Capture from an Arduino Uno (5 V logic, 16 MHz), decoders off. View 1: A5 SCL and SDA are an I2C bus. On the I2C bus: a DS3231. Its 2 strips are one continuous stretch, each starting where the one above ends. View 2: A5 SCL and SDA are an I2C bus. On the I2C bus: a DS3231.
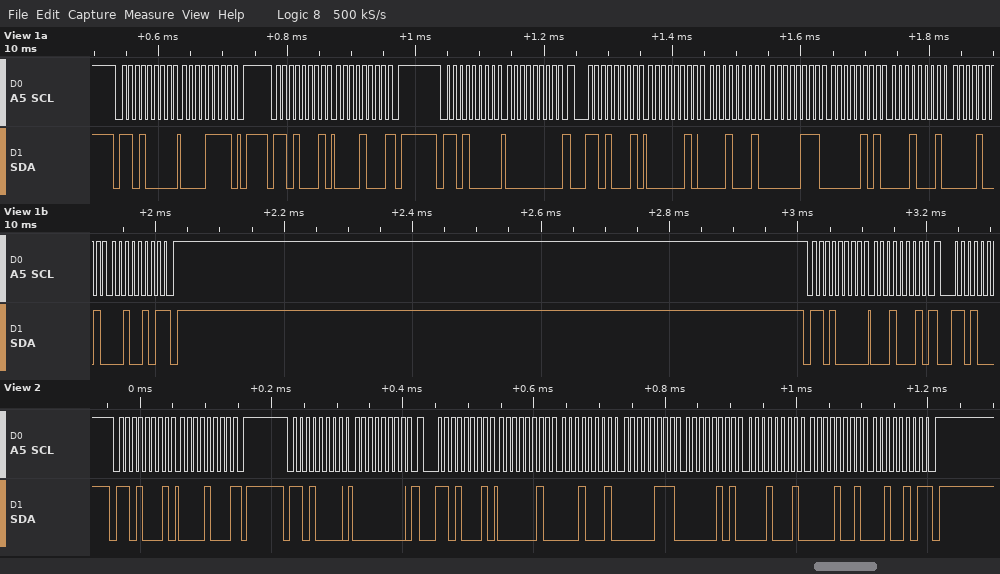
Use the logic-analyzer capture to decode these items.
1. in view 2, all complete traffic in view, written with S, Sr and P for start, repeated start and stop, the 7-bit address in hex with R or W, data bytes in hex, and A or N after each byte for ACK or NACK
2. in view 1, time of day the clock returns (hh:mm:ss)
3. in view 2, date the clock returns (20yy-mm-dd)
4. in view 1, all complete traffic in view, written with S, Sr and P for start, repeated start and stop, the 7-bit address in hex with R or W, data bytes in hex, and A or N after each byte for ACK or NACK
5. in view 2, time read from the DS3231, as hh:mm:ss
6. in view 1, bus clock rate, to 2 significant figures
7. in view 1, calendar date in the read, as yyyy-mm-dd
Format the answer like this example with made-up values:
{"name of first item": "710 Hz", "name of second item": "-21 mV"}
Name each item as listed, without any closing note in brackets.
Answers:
{"in view 2, all complete traffic in view, written with S, Sr and P for start, repeated start and stop, the 7-bit address in hex with R or W, data bytes in hex, and A or N after each byte for ACK or NACK": "S 68R A 08 N P S 68W A 00 A Sr 68R A 02 A 11 A 07 A 05 A 11 A 09 A 25 N P", "in view 1, time of day the clock returns": "07:11:02", "in view 2, date the clock returns": "2025-09-11", "in view 1, all complete traffic in view, written with S, Sr and P for start, repeated start and stop, the 7-bit address in hex with R or W, data bytes in hex, and A or N after each byte for ACK or NACK": "S 68W A 0F A P S 68R A 08 N P S 68W A 00 A Sr 68R A 02 A 11 A 07 A 05 A 11 A 09 A 25 N P S 68W A 11 A", "in view 2, time read from the DS3231, as hh:mm:ss": "07:11:02", "in view 1, bus clock rate, to 2 significant figures": "100 kHz", "in view 1, calendar date in the read, as yyyy-mm-dd": "2025-09-11"}
